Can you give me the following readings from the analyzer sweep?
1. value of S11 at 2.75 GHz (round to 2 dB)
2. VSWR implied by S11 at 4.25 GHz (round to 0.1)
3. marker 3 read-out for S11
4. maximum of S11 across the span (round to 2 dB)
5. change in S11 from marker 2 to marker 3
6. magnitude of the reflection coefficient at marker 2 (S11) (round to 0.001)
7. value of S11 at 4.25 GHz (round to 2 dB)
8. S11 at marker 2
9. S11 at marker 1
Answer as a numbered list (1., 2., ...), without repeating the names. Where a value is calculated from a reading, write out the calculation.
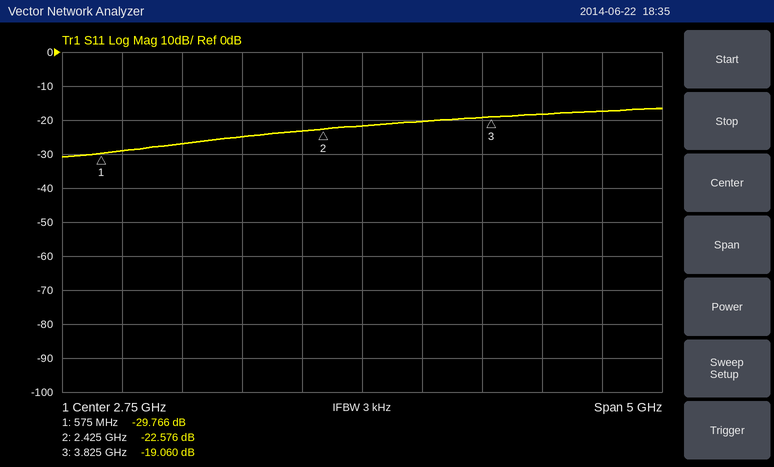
1. -22 dB
2. |Γ| = 10^(-18/20) = 0.1259; VSWR = (1 + 0.1259)/(1 − 0.1259) ≈ 1.3
3. -19.060 dB
4. -16 dB
5. -19.06 − (-22.576) = 3.516 dB
6. 10^(-22.576/20) ≈ 0.074
7. -18 dB
8. -22.576 dB
9. -29.766 dB
